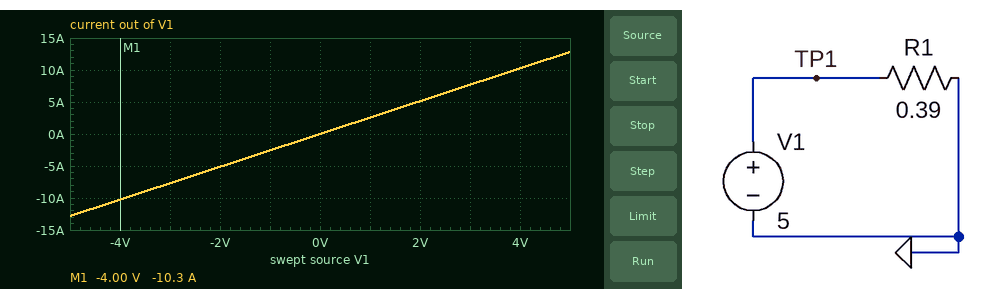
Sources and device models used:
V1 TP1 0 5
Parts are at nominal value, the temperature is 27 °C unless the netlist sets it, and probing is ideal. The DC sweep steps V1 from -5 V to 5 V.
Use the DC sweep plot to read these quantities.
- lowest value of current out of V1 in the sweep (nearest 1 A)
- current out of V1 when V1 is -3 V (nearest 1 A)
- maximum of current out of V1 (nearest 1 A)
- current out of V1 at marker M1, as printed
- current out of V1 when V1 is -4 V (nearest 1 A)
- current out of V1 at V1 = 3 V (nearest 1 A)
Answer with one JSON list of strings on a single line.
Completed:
["-13 A", "-8 A", "13 A", "-10.3 A", "-10 A", "8 A"]
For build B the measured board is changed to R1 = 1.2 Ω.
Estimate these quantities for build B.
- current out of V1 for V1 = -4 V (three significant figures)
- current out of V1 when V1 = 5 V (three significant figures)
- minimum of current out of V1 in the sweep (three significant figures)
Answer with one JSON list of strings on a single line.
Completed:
["-3.33 A", "4.17 A", "-4.17 A"]
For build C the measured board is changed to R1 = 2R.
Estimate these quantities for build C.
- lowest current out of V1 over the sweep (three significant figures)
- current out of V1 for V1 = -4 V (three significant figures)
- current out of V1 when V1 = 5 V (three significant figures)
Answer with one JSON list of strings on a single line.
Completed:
["-2.50 A", "-2.00 A", "2.50 A"]
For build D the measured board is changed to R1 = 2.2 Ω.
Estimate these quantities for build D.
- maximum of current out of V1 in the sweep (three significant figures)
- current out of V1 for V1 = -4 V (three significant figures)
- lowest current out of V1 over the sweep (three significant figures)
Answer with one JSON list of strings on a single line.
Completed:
["2.27 A", "-1.82 A", "-2.27 A"]
